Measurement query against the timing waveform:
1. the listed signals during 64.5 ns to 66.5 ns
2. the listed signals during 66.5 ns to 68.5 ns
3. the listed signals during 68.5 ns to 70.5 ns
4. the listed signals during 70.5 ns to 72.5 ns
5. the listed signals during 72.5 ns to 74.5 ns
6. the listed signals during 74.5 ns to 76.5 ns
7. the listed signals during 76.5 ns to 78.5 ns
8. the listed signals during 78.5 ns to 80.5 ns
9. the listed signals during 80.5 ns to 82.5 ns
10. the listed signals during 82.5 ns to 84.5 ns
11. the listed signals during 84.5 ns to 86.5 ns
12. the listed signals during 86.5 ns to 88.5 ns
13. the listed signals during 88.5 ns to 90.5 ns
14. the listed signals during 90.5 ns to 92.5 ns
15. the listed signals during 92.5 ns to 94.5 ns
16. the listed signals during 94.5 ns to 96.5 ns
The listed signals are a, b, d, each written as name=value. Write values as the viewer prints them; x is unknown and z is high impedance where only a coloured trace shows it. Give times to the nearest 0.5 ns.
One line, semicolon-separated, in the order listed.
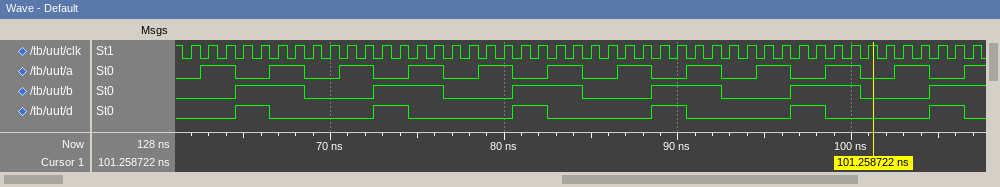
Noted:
a=0, b=1, d=1; a=1, b=1, d=0; a=0, b=0, d=0; a=1, b=0, d=0; a=0, b=1, d=1; a=1, b=1, d=0; a=0, b=0, d=0; a=1, b=0, d=0; a=0, b=1, d=1; a=1, b=1, d=0; a=0, b=0, d=0; a=1, b=0, d=0; a=0, b=1, d=1; a=1, b=1, d=0; a=0, b=0, d=0; a=1, b=0, d=0
